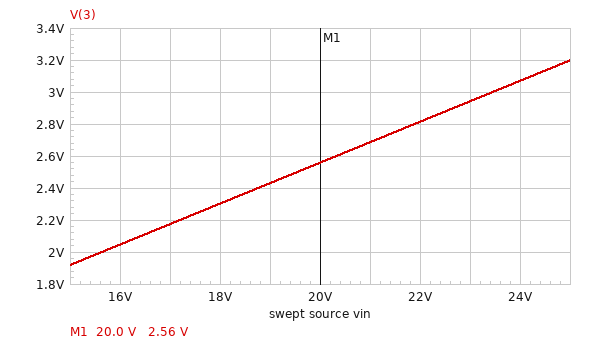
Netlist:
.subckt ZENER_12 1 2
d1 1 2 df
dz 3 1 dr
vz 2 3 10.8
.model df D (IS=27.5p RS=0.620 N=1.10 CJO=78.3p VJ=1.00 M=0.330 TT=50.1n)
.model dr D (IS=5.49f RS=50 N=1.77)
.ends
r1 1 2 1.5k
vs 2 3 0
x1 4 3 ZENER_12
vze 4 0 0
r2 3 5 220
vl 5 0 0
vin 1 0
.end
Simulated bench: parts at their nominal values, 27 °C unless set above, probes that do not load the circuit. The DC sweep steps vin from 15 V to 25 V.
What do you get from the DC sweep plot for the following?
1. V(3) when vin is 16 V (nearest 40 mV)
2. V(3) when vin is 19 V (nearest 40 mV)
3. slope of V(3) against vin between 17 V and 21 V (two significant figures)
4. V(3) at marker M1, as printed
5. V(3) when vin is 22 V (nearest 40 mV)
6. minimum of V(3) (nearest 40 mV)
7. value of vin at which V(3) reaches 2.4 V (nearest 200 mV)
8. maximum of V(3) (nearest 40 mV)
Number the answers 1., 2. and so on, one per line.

1. 2.04 V
2. 2.44 V
3. 0.13 V/V
4. 2.56 V
5. 2.80 V
6. 1.92 V
7. 18.8 V
8. 3.20 V
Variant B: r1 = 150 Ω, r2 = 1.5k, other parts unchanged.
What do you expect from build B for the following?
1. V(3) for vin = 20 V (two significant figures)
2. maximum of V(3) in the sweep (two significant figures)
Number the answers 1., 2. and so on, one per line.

1. 14 V
2. 15 V
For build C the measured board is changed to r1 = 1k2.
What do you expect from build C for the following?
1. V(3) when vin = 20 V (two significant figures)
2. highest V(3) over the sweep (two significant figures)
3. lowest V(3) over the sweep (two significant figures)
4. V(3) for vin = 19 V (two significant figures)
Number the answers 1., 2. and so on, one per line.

1. 3.1 V
2. 3.9 V
3. 2.3 V
4. 2.9 V
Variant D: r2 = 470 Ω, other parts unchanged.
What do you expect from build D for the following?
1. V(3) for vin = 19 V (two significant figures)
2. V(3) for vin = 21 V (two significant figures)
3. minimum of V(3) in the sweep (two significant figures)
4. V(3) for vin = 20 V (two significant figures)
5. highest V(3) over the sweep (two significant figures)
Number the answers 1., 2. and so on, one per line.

1. 4.5 V
2. 5.0 V
3. 3.6 V
4. 4.8 V
5. 6.0 V
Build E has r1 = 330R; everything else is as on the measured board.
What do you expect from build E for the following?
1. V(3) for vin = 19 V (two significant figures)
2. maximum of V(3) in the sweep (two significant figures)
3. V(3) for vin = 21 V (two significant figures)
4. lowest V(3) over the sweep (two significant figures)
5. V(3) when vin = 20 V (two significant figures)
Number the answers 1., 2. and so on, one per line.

1. 7.6 V
2. 10 V
3. 8.4 V
4. 6.0 V
5. 8.0 V
